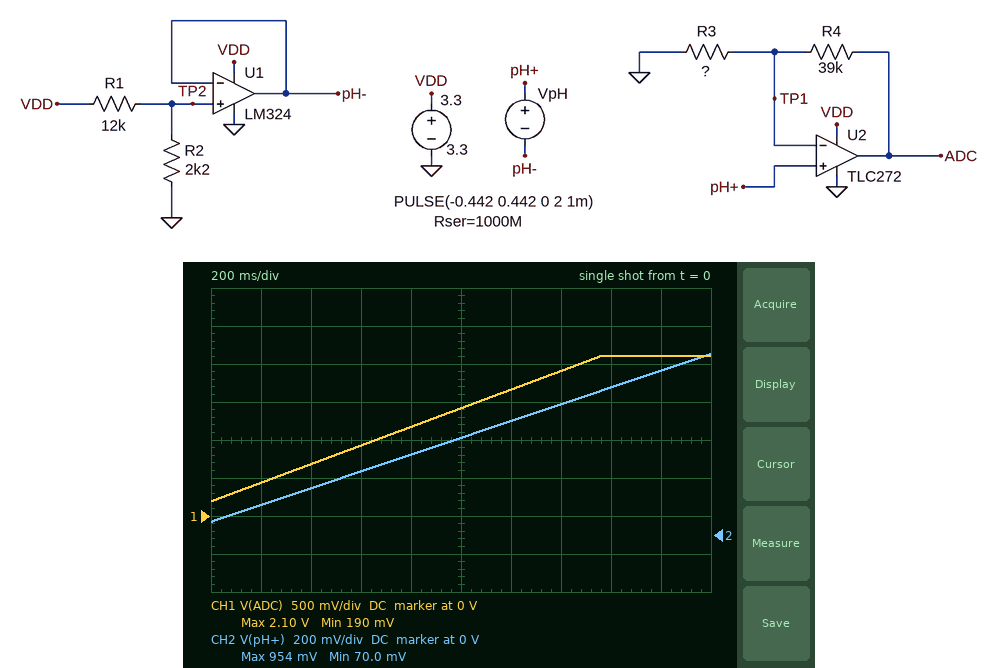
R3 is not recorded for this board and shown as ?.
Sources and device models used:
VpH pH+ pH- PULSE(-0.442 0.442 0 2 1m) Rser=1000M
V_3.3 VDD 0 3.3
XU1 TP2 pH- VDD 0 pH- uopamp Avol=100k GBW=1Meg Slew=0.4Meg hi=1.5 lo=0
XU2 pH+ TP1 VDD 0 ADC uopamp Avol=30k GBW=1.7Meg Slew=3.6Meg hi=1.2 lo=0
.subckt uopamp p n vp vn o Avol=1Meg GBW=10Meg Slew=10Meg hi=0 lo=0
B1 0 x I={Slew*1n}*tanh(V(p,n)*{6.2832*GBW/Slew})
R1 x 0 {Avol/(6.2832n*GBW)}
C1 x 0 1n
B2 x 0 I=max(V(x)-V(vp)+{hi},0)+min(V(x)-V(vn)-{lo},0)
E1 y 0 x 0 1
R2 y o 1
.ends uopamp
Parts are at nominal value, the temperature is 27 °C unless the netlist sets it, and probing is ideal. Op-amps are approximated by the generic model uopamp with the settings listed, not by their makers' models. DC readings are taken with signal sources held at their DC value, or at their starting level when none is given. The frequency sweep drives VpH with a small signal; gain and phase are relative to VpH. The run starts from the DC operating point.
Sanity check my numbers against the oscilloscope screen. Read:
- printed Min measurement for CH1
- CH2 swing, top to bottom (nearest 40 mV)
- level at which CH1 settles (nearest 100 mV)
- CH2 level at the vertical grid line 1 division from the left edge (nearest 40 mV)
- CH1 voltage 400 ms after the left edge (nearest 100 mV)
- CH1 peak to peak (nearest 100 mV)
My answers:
190 mV
880 mV
2.1 V
160 mV
700 mV
1.9 V
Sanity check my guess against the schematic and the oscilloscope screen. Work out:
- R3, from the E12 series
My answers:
22 kΩ
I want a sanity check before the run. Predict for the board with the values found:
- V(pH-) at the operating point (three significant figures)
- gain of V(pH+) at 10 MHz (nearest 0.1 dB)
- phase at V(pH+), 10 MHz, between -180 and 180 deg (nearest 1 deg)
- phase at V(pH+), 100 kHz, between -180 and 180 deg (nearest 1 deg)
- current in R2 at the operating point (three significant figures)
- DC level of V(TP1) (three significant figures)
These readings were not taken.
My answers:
511 mV
0 dB
0 deg
0 deg
232 µA
69.3 mV
